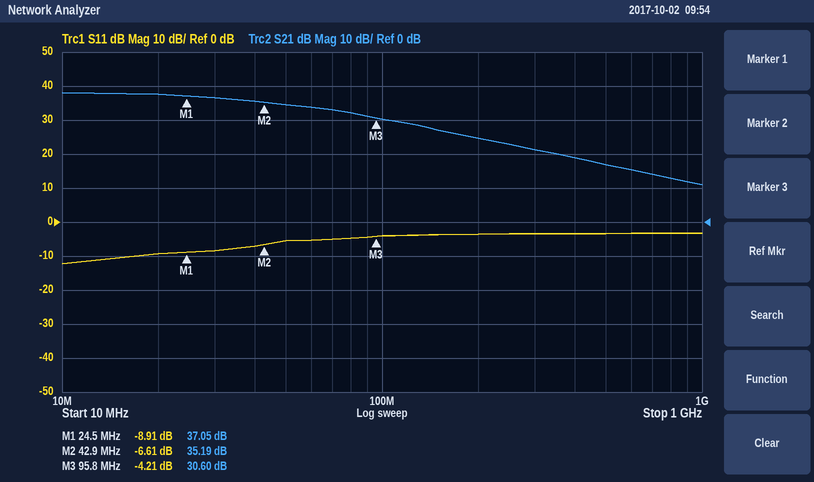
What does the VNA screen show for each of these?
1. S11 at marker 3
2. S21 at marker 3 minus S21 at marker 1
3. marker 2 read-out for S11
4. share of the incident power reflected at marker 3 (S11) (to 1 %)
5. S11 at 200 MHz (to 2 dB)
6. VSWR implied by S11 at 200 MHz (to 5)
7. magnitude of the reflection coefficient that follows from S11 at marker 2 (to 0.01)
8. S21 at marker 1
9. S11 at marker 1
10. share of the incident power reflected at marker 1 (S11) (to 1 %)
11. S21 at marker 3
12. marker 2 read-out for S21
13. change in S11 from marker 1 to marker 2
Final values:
-4.21 dB
-6.45 dB
-6.61 dB
38 %
-4 dB
5
0.47
37.05 dB
-8.91 dB
13 %
30.60 dB
35.19 dB
2.30 dB
